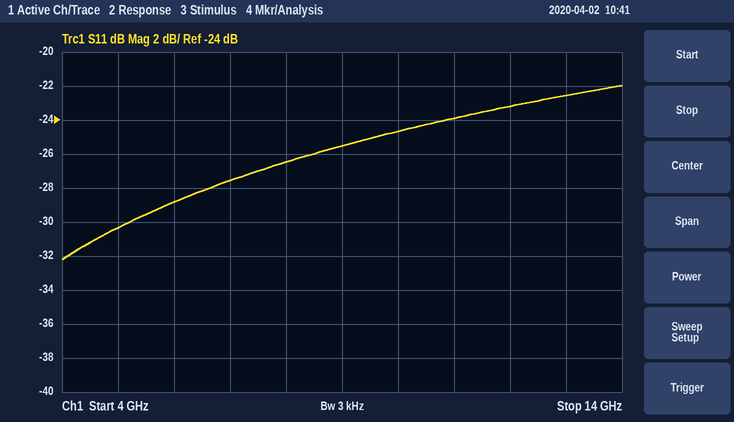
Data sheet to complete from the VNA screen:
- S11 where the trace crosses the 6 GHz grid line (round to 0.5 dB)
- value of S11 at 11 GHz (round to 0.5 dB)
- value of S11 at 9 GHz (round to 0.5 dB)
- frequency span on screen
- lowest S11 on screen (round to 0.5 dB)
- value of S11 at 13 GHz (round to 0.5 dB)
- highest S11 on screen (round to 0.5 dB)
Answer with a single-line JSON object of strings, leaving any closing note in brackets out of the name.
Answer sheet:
{"S11 where the trace crosses the 6 GHz grid line": "-29.0 dB", "value of S11 at 11 GHz": "-24.0 dB", "value of S11 at 9 GHz": "-25.5 dB", "frequency span on screen": "10 GHz", "lowest S11 on screen": "-32.0 dB", "value of S11 at 13 GHz": "-22.5 dB", "highest S11 on screen": "-22.0 dB"}
